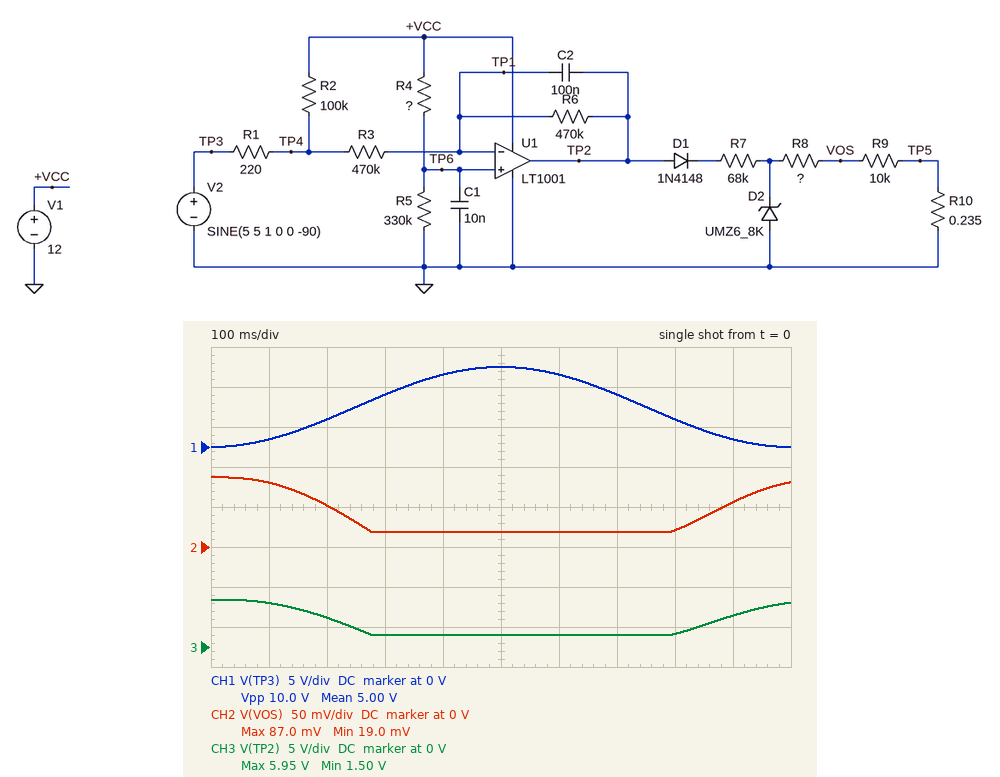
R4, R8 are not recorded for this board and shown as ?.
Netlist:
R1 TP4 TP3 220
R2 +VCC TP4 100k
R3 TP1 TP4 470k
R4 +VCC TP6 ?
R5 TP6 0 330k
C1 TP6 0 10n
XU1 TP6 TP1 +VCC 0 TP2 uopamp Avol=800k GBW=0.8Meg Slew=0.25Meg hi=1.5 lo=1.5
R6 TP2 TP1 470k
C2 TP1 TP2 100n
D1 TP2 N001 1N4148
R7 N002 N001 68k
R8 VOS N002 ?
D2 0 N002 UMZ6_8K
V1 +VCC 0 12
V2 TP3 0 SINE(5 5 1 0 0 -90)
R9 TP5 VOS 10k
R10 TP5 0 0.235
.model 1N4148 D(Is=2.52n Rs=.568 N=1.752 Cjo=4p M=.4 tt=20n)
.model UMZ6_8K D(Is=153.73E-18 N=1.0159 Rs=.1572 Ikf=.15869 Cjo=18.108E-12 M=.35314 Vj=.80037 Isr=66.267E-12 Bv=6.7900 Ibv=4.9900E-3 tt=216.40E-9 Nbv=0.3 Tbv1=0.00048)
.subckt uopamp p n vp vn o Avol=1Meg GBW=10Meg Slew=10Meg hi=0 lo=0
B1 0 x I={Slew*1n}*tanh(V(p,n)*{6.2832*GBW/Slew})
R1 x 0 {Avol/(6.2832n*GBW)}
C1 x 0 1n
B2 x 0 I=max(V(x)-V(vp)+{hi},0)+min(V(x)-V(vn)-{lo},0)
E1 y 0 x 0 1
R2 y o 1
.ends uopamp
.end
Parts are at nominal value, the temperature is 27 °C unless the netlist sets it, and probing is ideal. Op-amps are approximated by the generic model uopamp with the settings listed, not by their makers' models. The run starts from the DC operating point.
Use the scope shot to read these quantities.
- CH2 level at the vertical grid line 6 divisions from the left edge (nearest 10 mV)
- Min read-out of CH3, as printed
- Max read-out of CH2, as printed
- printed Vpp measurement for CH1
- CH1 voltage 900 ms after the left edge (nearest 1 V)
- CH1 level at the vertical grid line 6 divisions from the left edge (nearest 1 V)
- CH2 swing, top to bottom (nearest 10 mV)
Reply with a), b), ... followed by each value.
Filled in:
a) 20 mV
b) 1.50 V
c) 87.0 mV
d) 10.0 V
e) 1 V
f) 9 V
g) 70 mV
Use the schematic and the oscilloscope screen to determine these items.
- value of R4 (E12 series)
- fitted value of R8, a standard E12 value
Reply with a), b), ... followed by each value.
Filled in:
a) 1 MΩ
b) 560 kΩ
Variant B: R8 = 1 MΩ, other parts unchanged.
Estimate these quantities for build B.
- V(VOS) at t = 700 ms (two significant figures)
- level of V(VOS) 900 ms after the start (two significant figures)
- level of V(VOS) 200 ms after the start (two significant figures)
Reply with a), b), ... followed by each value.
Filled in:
a) 11 mV
b) 33 mV
c) 31 mV
